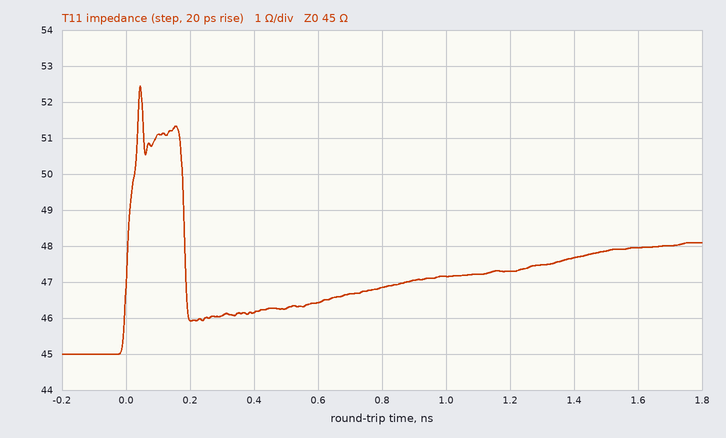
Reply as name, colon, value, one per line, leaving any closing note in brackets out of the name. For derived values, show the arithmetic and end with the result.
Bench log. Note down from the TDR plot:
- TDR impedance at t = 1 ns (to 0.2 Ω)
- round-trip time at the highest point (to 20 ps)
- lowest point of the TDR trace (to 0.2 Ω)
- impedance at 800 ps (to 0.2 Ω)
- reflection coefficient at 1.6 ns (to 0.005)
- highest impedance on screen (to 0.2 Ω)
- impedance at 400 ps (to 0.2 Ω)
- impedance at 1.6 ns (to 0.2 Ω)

TDR impedance at t = 1 ns: 47.2 Ω
round-trip time at the highest point: 40 ps
lowest point of the TDR trace: 45.0 Ω
impedance at 800 ps: 46.8 Ω
reflection coefficient at 1.6 ns: (48 − 45)/(48 + 45) ≈ +0.0323, so +0.030 to the nearest 0.005
highest impedance on screen: 52.4 Ω
impedance at 400 ps: 46.2 Ω
impedance at 1.6 ns: 48.0 Ω
